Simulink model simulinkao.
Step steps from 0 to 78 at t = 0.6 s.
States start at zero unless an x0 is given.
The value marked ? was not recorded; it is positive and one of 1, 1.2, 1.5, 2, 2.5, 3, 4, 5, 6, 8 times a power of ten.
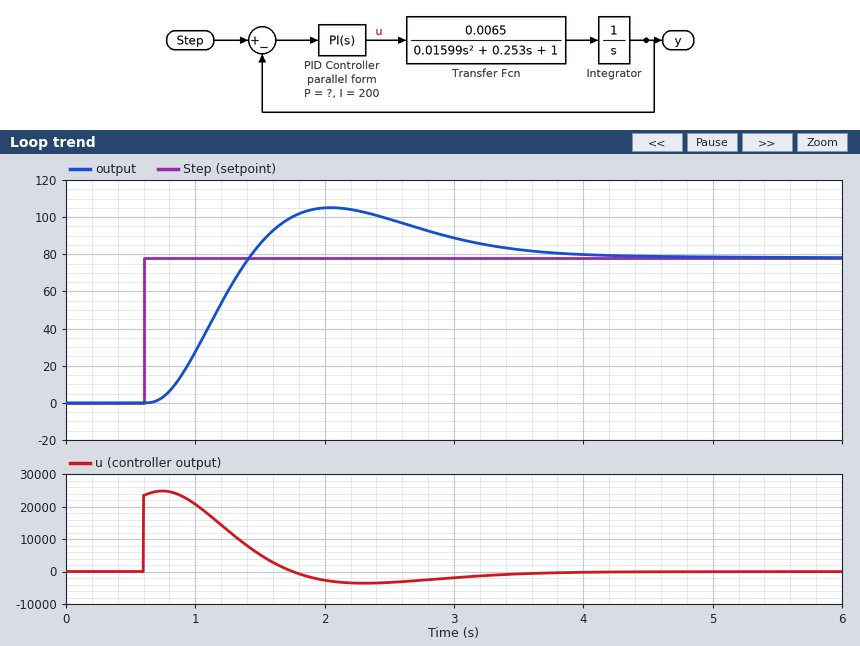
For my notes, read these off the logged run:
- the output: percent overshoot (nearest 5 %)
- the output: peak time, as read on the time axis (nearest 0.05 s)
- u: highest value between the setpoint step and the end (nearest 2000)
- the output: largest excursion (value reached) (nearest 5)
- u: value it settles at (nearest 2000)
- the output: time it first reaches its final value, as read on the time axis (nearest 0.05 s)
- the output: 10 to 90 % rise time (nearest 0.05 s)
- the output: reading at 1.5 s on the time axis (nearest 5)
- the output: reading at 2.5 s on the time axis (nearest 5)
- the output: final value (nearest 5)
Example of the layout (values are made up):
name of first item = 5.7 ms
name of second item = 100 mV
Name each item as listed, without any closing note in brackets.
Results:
the output: percent overshoot = 35 %
the output: peak time, as read on the time axis = 2.05 s
u: highest value between the setpoint step and the end = 24000
the output: largest excursion (value reached) = 105
u: value it settles at = 0
the output: time it first reaches its final value, as read on the time axis = 1.40 s
the output: 10 to 90 % rise time = 0.50 s
the output: reading at 1.5 s on the time axis = 85
the output: reading at 2.5 s on the time axis = 100
the output: final value = 80
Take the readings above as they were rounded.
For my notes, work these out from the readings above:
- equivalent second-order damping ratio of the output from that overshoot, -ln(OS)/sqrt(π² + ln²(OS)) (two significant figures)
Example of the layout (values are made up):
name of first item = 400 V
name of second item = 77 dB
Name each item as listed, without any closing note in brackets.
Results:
equivalent second-order damping ratio of the output from that overshoot, -ln(OS)/sqrt(π² + ln²(OS)) = 0.32
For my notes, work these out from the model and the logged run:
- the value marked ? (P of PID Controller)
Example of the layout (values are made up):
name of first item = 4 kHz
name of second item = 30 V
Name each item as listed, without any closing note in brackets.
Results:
the value marked ? = 300
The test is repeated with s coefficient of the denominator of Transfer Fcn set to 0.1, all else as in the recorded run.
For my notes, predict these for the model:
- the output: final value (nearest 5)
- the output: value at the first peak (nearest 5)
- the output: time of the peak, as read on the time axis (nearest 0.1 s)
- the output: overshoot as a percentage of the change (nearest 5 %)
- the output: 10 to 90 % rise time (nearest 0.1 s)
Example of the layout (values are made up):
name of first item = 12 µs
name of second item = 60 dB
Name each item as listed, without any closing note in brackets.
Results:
the output: final value = 80
the output: value at the first peak = 95
the output: time of the peak, as read on the time axis = 2.2 s
the output: overshoot as a percentage of the change = 20 %
the output: 10 to 90 % rise time = 0.4 s
